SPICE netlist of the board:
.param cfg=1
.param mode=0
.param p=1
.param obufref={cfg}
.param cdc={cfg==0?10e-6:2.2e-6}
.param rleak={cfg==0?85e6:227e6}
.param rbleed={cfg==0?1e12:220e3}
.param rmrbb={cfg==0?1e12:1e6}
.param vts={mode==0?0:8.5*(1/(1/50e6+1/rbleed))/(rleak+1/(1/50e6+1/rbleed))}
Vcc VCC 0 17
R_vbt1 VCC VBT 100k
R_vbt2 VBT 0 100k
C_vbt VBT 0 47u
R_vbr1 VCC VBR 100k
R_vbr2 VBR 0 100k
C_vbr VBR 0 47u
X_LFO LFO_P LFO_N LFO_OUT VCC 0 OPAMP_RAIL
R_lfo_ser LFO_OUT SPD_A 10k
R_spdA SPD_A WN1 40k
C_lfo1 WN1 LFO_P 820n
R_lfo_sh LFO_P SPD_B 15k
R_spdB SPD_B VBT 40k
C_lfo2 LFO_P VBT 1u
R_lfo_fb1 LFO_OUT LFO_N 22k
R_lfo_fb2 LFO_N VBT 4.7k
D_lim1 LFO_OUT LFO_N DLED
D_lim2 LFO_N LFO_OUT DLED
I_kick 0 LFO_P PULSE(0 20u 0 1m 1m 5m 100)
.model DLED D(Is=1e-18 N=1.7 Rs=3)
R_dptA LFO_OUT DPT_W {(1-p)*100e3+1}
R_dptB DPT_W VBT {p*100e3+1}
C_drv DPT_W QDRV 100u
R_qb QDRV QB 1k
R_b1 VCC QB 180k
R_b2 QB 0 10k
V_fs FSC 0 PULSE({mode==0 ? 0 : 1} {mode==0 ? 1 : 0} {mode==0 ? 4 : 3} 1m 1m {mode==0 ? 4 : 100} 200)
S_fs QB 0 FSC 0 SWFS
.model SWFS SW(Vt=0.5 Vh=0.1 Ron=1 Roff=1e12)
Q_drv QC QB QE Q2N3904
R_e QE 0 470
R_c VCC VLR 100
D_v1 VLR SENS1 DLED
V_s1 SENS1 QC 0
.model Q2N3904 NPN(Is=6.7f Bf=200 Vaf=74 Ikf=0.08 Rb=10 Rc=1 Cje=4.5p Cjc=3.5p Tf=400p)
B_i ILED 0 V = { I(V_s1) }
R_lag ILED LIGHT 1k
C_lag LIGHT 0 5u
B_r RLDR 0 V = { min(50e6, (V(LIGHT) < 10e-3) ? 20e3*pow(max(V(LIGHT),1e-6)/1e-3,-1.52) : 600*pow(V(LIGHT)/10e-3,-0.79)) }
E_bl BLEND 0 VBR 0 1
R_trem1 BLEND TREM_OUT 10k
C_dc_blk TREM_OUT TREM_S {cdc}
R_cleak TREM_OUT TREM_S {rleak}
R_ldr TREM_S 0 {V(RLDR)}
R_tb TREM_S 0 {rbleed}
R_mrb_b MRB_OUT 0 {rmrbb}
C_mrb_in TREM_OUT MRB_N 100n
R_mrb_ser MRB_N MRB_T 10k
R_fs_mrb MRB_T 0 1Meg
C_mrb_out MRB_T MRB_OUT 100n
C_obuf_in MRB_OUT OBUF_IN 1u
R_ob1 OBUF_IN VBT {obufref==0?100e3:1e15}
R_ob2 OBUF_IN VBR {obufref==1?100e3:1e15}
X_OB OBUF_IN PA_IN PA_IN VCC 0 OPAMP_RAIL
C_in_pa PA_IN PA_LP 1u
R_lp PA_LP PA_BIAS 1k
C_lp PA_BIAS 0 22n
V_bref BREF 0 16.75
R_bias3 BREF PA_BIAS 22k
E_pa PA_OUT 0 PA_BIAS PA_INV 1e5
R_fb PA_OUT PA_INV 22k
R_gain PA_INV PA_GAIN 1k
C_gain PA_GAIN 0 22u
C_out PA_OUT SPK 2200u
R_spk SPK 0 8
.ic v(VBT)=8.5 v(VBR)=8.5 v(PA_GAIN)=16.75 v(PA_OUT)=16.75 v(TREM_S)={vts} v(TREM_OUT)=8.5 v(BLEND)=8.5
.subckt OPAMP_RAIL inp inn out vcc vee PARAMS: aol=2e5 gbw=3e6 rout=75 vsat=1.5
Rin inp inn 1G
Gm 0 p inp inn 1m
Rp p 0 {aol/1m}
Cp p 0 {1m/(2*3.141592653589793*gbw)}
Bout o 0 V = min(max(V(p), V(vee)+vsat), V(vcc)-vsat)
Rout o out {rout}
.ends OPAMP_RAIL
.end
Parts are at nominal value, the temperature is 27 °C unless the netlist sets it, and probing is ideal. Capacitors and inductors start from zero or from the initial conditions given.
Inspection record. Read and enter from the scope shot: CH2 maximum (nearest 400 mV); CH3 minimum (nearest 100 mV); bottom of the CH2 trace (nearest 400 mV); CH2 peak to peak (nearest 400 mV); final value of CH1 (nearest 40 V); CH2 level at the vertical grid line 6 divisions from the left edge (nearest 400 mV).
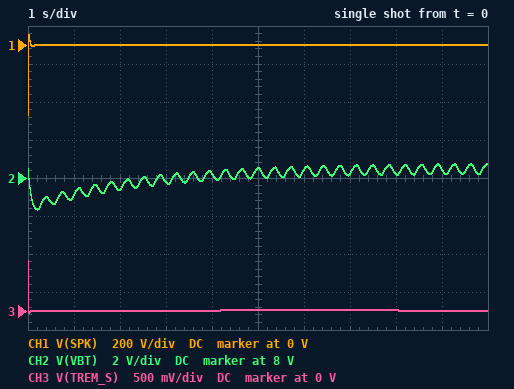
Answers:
8.8 V
0 V
6.4 V
2.4 V
0 V
8.4 V
